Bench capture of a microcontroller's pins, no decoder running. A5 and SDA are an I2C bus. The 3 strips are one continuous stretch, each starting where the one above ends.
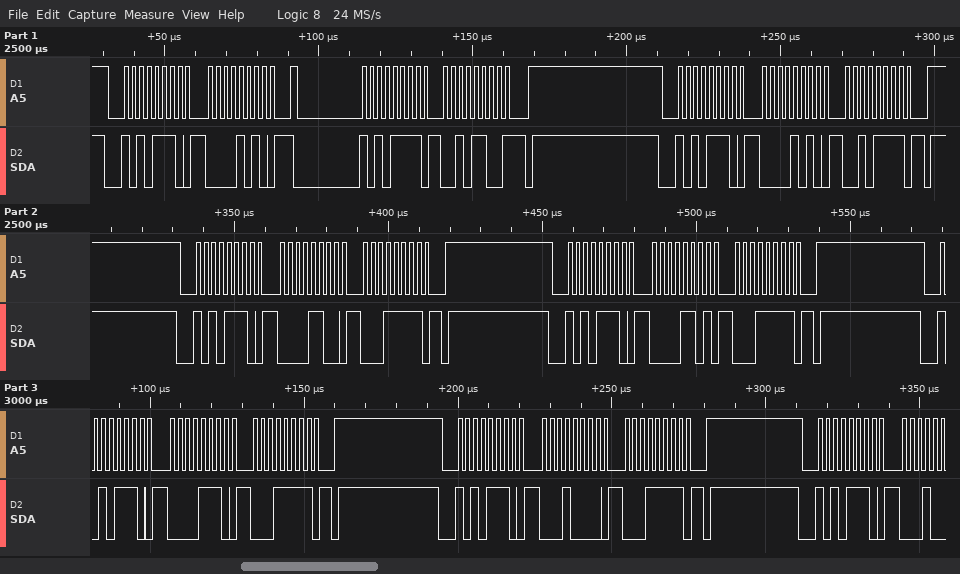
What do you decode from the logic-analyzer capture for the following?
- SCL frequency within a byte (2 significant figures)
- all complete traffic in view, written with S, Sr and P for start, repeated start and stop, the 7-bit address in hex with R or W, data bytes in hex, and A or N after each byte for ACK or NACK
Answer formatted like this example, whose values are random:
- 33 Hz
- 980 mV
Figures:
- 400 kHz
- S 57W A 0A A Sr 57R A 2C N P S 57W A 0A A 2F A P S 57W A 0C A 1F A P S 57W A 0D A 1F A P S 57W A 0E A 1F A P S 57W A 10 A 1F A P S 57W A
